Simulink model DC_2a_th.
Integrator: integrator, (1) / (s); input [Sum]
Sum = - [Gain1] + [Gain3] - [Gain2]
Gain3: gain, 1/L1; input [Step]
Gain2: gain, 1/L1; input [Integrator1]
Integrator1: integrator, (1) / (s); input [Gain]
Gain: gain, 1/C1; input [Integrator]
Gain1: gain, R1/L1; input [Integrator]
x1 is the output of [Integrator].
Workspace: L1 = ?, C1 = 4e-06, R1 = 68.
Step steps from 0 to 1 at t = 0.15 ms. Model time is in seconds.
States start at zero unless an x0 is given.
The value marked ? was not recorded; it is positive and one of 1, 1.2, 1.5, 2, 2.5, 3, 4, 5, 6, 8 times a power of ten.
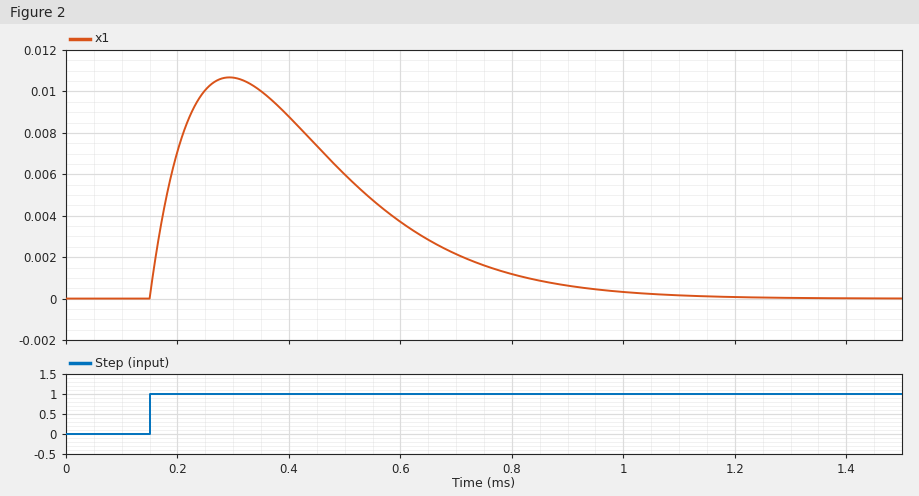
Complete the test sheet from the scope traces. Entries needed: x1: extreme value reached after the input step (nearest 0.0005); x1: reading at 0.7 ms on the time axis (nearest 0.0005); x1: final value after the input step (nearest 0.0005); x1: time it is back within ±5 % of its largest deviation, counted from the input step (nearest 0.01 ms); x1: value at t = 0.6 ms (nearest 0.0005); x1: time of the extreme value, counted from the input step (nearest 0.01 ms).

0.0105
0.0020
0.0000
0.77 ms
0.0035
0.14 ms
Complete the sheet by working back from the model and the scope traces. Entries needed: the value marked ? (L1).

0.005
